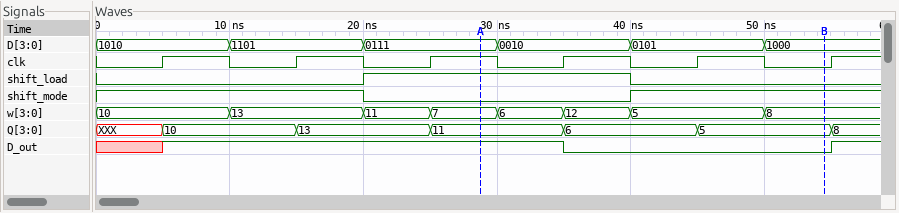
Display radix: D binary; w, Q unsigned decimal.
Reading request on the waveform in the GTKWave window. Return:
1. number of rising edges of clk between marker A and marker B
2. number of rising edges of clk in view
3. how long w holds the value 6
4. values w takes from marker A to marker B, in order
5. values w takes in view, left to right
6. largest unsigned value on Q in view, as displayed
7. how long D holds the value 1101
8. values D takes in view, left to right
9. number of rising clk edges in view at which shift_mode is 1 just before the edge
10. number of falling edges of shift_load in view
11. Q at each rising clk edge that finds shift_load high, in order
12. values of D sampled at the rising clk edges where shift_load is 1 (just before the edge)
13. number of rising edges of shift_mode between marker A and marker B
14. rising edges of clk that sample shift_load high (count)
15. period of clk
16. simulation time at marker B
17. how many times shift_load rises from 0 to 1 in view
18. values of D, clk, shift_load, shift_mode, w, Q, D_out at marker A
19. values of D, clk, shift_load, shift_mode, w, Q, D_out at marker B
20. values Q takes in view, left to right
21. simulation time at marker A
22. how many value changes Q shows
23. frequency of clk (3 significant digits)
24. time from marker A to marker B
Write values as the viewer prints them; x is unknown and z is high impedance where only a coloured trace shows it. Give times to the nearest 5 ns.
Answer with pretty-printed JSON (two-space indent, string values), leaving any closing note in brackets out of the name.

{
  "number of rising edges of clk between marker A and marker B": "2",
  "number of rising edges of clk in view": "6",
  "how long w holds the value 6": "5 ns",
  "values w takes from marker A to marker B, in order": "7, 6, 12, 5, 8",
  "values w takes in view, left to right": "10, 13, 11, 7, 6, 12, 5, 8",
  "largest unsigned value on Q in view, as displayed": "13",
  "how long D holds the value 1101": "10 ns",
  "values D takes in view, left to right": "1010, 1101, 0111, 0010, 0101, 1000",
  "number of rising clk edges in view at which shift_mode is 1 just before the edge": "4",
  "number of falling edges of shift_load in view": "1",
  "Q at each rising clk edge that finds shift_load high, in order": "13, 11",
  "values of D sampled at the rising clk edges where shift_load is 1": "0111, 0010",
  "number of rising edges of shift_mode between marker A and marker B": "1",
  "rising edges of clk that sample shift_load high": "2",
  "period of clk": "10 ns",
  "simulation time at marker B": "55 ns",
  "how many times shift_load rises from 0 to 1 in view": "1",
  "values of D, clk, shift_load, shift_mode, w, Q, D_out at marker A": "D=0111, clk=1, shift_load=1, shift_mode=0, w=7, Q=11, D_out=1",
  "values of D, clk, shift_load, shift_mode, w, Q, D_out at marker B": "D=1000, clk=0, shift_load=0, shift_mode=1, w=8, Q=5, D_out=0",
  "values Q takes in view, left to right": "XXX, 10, 13, 11, 6, 5, 8",
  "simulation time at marker A": "30 ns",
  "how many value changes Q shows": "6",
  "frequency of clk": "100 MHz",
  "time from marker A to marker B": "25 ns"
}
